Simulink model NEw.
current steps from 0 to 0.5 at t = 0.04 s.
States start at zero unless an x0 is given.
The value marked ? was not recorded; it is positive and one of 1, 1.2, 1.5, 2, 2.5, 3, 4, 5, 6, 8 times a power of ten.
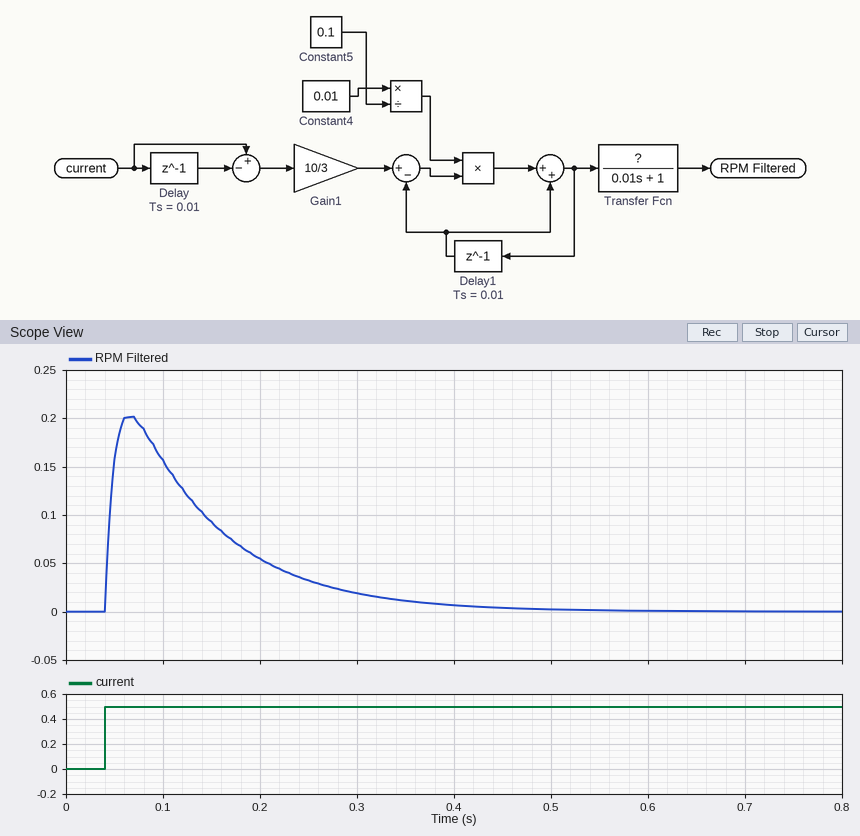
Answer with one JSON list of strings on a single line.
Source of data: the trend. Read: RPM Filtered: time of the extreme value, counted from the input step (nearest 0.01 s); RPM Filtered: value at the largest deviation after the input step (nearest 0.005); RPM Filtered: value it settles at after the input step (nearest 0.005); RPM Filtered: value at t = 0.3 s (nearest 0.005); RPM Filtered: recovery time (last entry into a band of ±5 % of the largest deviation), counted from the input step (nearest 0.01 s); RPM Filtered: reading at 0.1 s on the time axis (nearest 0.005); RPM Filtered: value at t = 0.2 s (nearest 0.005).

["0.03 s", "0.200", "0.000", "0.020", "0.32 s", "0.155", "0.055"]
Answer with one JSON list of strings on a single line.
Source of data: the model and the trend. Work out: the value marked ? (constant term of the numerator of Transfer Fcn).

["1.5"]
